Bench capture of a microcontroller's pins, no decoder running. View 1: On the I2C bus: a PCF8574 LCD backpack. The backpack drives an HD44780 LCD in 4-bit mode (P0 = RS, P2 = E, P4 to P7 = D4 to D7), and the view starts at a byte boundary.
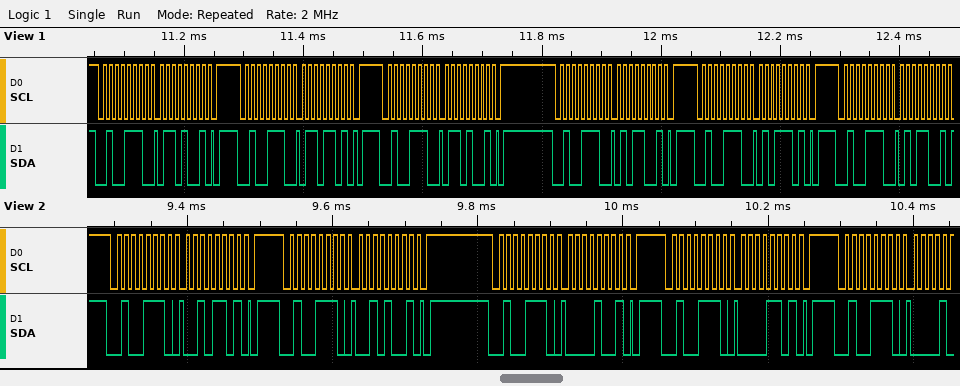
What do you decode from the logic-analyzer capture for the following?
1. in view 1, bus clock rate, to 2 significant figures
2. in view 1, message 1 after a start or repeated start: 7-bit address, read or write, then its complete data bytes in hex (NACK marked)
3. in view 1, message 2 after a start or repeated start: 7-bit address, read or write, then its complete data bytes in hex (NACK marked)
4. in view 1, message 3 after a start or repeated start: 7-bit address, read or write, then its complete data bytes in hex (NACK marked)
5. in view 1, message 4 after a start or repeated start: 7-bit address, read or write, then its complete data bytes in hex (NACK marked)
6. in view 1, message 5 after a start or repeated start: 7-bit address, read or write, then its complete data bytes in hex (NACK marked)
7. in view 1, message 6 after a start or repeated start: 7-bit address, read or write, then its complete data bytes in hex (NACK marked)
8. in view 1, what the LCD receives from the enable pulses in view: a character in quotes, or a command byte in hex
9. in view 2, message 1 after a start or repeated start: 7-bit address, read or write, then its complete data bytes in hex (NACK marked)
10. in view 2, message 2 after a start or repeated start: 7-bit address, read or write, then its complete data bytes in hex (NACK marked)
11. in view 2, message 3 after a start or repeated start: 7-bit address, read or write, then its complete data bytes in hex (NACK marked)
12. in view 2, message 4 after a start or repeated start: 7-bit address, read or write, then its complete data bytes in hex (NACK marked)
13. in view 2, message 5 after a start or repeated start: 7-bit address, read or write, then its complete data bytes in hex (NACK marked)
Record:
100 kHz
0x27 write: 69
0x27 write: 6D
0x27 write: 69
0x27 write: 59
0x27 write: 5D
0x27 write: 59
'e'
0x27 write: 2D
0x27 write: 29
0x27 write: 09
0x27 write: 0D
0x27 write
